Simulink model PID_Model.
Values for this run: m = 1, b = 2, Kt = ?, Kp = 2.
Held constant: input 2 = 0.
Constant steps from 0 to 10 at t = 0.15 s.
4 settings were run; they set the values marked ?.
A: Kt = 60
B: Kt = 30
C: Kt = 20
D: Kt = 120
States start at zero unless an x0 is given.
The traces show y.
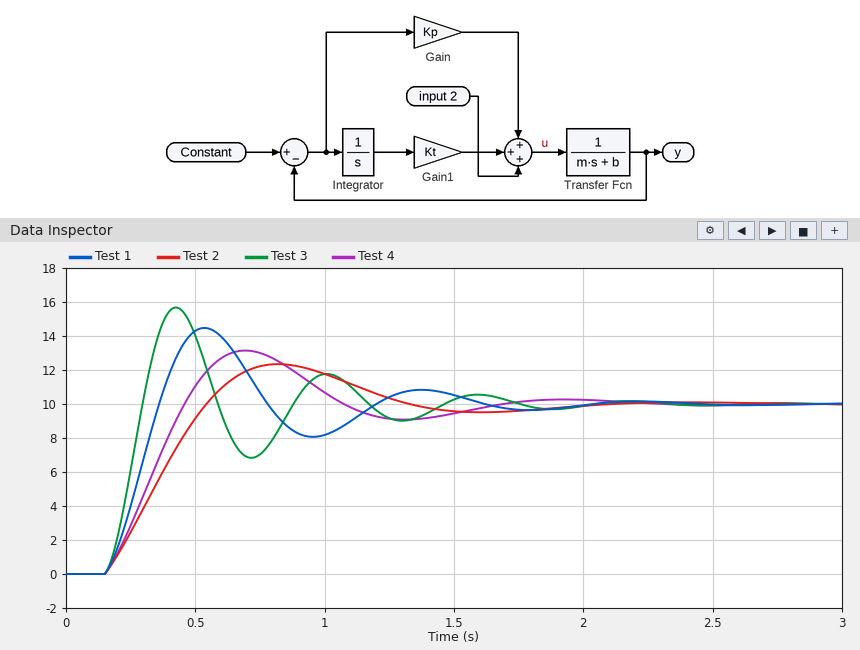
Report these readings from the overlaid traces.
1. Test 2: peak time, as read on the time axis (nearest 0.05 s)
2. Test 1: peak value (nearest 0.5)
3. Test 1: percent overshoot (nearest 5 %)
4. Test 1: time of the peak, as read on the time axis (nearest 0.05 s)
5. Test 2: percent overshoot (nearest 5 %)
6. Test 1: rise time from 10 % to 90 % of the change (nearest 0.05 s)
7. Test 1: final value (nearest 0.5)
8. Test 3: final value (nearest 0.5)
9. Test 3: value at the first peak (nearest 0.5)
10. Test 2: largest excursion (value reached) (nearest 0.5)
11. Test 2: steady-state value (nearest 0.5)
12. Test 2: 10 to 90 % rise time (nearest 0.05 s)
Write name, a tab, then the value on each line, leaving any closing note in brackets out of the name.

Test 2: peak time, as read on the time axis	0.80 s
Test 1: peak value	14.5
Test 1: percent overshoot	45 %
Test 1: time of the peak, as read on the time axis	0.55 s
Test 2: percent overshoot	25 %
Test 1: rise time from 10 % to 90 % of the change	0.15 s
Test 1: final value	10.0
Test 3: final value	10.0
Test 3: value at the first peak	15.5
Test 2: largest excursion (value reached)	12.5
Test 2: steady-state value	10.0
Test 2: 10 to 90 % rise time	0.30 s
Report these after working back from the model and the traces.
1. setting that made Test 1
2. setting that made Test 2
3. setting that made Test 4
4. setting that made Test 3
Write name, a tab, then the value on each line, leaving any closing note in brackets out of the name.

setting that made Test 1	A
setting that made Test 2	C
setting that made Test 4	B
setting that made Test 3	D
